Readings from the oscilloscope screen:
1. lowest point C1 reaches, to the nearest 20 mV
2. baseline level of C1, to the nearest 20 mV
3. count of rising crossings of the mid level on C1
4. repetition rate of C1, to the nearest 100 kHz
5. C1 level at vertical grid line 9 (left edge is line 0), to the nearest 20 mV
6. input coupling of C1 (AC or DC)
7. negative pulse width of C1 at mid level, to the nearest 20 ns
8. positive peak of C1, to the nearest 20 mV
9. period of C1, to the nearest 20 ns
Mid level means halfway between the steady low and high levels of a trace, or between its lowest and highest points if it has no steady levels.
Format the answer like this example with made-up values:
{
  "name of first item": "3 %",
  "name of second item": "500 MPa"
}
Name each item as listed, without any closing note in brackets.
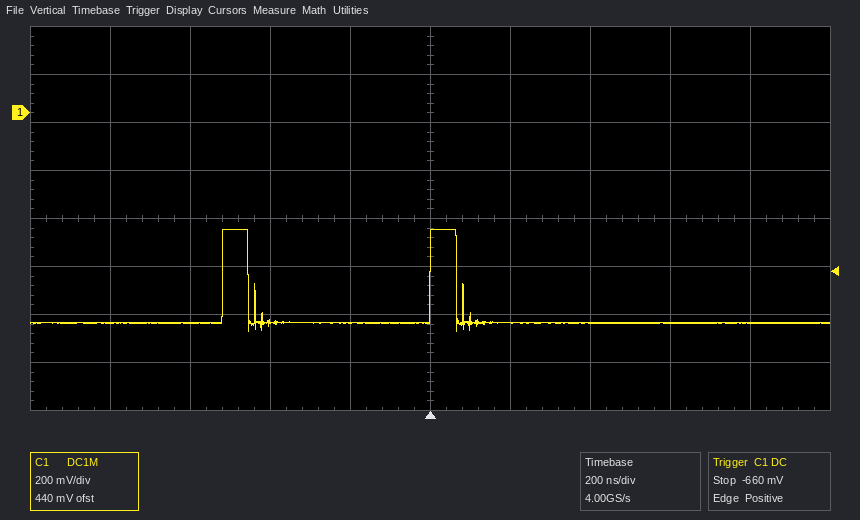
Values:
{
  "lowest point C1 reaches, to the nearest 20 mV": "-920 mV",
  "baseline level of C1, to the nearest 20 mV": "-880 mV",
  "count of rising crossings of the mid level on C1": "2",
  "repetition rate of C1, to the nearest 100 kHz": "1.9 MHz",
  "C1 level at vertical grid line 9 (left edge is line 0), to the nearest 20 mV": "-880 mV",
  "input coupling of C1": "DC",
  "negative pulse width of C1 at mid level, to the nearest 20 ns": "460 ns",
  "positive peak of C1, to the nearest 20 mV": "-480 mV",
  "period of C1, to the nearest 20 ns": "520 ns"
}
